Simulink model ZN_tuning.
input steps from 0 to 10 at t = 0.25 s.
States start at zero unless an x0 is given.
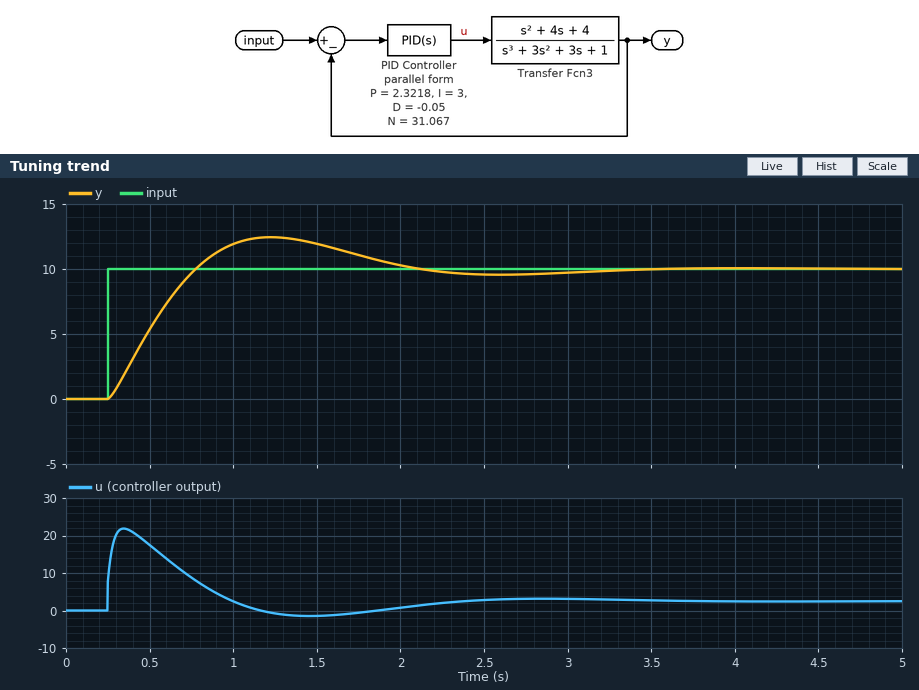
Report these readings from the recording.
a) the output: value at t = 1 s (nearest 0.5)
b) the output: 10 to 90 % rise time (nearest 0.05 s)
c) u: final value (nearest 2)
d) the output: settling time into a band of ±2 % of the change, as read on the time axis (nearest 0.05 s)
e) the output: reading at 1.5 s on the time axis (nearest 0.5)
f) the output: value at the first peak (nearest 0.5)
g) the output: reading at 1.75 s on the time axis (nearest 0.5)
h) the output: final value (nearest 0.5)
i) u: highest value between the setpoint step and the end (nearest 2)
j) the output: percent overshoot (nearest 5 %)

12.0
0.40 s
2
3.15 s
12.0
12.5
11.0
10.0
22
25 %
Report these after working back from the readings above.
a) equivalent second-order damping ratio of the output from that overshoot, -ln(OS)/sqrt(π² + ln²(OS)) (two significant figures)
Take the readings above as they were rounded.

0.40
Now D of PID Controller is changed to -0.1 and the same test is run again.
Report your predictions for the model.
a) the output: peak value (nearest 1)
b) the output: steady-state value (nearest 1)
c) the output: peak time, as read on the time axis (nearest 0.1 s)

13
10
1.2 s
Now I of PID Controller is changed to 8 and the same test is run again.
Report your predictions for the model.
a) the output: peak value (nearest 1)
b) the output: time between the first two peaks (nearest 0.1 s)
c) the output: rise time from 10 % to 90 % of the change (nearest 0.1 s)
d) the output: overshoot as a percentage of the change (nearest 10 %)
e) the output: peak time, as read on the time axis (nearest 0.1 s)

14
1.9 s
0.3 s
40 %
1.0 s
